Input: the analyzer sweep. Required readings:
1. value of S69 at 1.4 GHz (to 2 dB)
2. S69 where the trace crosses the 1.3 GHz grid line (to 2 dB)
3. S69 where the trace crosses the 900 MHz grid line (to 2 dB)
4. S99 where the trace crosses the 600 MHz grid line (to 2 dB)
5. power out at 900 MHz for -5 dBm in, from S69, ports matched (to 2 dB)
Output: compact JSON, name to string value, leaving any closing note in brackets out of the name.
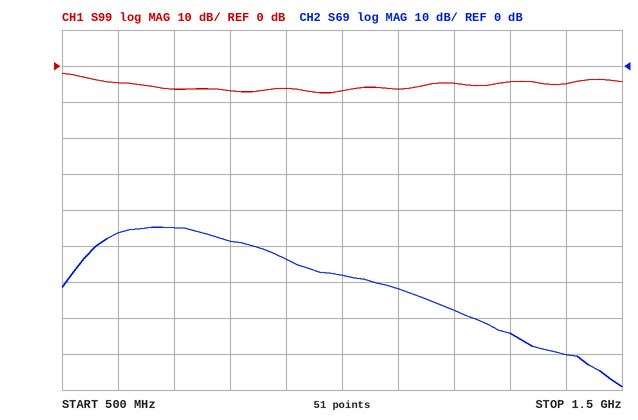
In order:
{"value of S69 at 1.4 GHz": "-80 dB", "S69 where the trace crosses the 1.3 GHz grid line": "-74 dB", "S69 where the trace crosses the 900 MHz grid line": "-54 dB", "S99 where the trace crosses the 600 MHz grid line": "-4 dB", "power out at 900 MHz for -5 dBm in, from S69, ports matched": "-58 dBm"}
